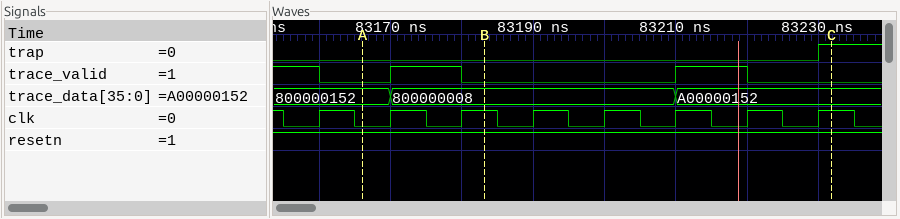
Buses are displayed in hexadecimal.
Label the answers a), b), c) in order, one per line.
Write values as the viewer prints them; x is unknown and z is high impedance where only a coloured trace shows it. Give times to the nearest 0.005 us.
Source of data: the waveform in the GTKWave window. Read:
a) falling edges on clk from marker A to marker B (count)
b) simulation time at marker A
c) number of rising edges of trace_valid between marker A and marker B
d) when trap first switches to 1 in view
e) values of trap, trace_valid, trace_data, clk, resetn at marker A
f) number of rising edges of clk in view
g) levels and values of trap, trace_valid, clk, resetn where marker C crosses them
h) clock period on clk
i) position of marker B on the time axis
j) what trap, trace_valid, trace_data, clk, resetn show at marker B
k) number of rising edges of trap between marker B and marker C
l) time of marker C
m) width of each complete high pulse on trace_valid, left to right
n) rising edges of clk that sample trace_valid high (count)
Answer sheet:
a) 1
b) 83.165 us
c) 1
d) 83.23 us
e) trap=0, trace_valid=0, trace_data=800000152, clk=0, resetn=1
f) 8
g) trap=1, trace_valid=0, clk=1, resetn=1
h) 0.01 us
i) 83.185 us
j) trap=0, trace_valid=0, trace_data=800000008, clk=1, resetn=1
k) 1
l) 83.23 us
m) 0.01 us, 0.01 us
n) 3
